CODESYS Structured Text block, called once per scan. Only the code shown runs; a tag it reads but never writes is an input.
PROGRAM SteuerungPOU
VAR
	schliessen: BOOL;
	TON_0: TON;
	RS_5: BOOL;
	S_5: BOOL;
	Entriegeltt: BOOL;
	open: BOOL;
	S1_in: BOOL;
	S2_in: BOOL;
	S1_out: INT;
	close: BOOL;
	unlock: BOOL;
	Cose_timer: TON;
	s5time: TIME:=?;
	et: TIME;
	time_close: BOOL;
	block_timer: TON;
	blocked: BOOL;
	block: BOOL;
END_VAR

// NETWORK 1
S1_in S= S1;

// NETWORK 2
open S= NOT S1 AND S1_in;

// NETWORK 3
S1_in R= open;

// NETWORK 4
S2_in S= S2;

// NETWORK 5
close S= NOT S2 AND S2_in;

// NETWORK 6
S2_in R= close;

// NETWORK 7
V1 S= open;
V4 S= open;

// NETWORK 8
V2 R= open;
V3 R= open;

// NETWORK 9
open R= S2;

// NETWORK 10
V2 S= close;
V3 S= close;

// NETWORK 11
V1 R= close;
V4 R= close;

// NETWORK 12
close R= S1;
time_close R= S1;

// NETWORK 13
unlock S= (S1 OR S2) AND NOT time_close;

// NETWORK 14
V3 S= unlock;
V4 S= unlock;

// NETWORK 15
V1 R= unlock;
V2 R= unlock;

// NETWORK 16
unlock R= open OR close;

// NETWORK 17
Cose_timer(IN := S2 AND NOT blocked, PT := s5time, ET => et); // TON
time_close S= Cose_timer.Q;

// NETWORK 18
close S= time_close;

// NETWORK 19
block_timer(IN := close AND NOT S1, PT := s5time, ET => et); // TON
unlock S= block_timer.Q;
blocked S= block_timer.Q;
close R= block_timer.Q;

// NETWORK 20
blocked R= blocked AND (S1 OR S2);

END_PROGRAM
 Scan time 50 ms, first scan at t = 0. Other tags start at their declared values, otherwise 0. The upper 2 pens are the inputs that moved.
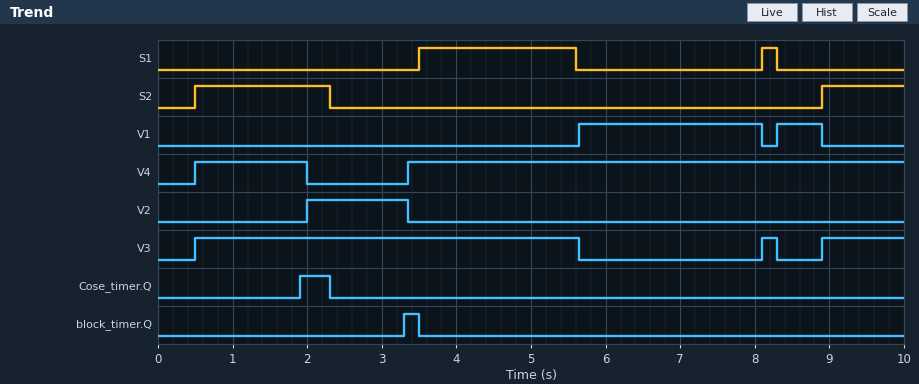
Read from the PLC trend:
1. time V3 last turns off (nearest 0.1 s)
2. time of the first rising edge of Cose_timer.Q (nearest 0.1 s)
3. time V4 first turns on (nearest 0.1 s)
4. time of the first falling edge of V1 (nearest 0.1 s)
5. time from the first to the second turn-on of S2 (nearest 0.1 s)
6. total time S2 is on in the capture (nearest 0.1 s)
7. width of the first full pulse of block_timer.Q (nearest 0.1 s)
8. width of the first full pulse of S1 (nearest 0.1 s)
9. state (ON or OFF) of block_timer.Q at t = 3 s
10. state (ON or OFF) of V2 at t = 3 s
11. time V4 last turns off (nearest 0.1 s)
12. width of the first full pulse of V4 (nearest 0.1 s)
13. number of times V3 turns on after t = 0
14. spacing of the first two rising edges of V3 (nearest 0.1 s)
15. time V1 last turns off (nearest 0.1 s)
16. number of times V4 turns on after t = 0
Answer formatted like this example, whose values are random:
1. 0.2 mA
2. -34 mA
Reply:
1. 8.3 s
2. 1.9 s
3. 0.5 s
4. 8.1 s
5. 8.4 s
6. 2.9 s
7. 0.2 s
8. 2.1 s
9. OFF
10. ON
11. 2.0 s
12. 1.5 s
13. 3
14. 7.6 s
15. 8.9 s
16. 2
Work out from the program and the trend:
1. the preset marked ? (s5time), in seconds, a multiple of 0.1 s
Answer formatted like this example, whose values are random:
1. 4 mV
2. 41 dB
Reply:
1. 1.4 s
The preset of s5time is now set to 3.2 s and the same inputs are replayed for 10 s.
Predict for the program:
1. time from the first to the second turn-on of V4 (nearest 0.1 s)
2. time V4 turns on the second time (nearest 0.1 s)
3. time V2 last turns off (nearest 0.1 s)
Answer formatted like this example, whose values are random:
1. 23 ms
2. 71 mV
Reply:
1. 3.0 s
2. 3.5 s
3. 3.5 s
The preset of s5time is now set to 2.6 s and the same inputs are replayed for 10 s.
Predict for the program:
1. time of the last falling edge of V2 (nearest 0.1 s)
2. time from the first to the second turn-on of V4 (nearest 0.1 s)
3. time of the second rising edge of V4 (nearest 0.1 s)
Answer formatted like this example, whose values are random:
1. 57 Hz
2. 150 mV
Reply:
1. 3.5 s
2. 3.0 s
3. 3.5 s
